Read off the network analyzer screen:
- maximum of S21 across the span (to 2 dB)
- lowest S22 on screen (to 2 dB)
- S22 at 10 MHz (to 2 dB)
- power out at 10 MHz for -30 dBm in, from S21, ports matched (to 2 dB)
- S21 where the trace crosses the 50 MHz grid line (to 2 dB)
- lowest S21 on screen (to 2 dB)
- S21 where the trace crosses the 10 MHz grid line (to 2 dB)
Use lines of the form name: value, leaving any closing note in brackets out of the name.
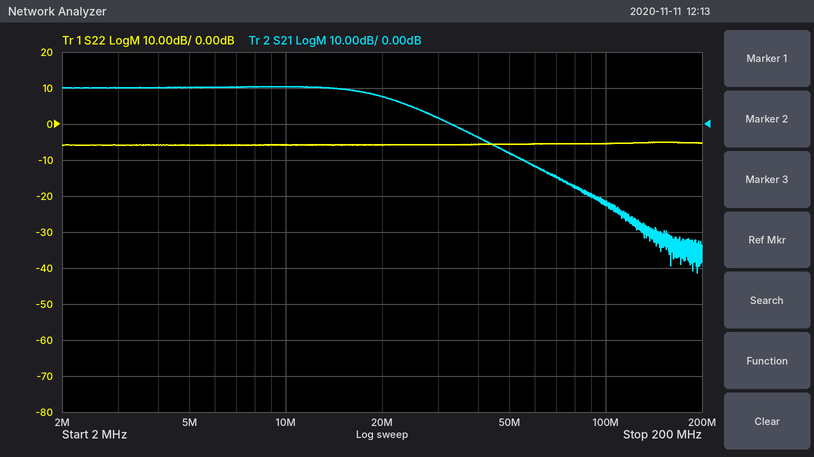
maximum of S21 across the span: 10 dB
lowest S22 on screen: -6 dB
S22 at 10 MHz: -6 dB
power out at 10 MHz for -30 dBm in, from S21, ports matched: -20 dBm
S21 where the trace crosses the 50 MHz grid line: -8 dB
lowest S21 on screen: -42 dB
S21 where the trace crosses the 10 MHz grid line: 10 dB
